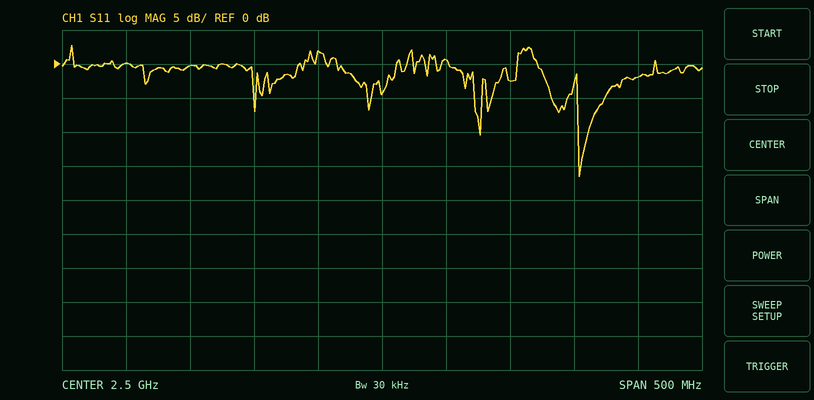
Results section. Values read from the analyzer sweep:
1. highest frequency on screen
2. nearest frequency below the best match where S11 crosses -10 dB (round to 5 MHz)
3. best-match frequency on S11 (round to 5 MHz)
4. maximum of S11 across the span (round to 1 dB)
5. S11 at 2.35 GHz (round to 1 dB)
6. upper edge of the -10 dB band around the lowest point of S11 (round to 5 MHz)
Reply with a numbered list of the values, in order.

1. 2.75 GHz
2. 2.655 GHz
3. 2.655 GHz
4. 3 dB
5. 0 dB
6. 2.660 GHz
